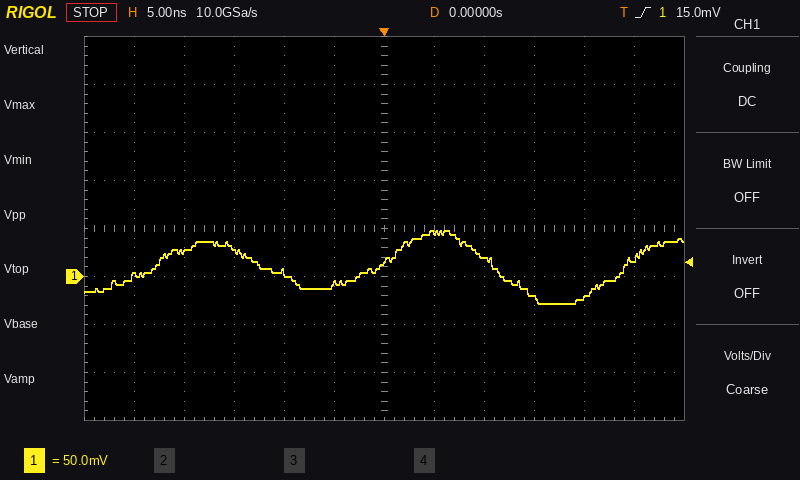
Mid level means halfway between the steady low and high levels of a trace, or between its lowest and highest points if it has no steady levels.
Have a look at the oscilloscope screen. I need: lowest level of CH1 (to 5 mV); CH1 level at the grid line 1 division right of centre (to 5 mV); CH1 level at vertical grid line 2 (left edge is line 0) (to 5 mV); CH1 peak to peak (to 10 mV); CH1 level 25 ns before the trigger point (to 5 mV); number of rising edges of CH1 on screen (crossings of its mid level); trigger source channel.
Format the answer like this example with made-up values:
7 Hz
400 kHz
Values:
-30 mV
45 mV
25 mV
80 mV
0 mV
3
CH1
